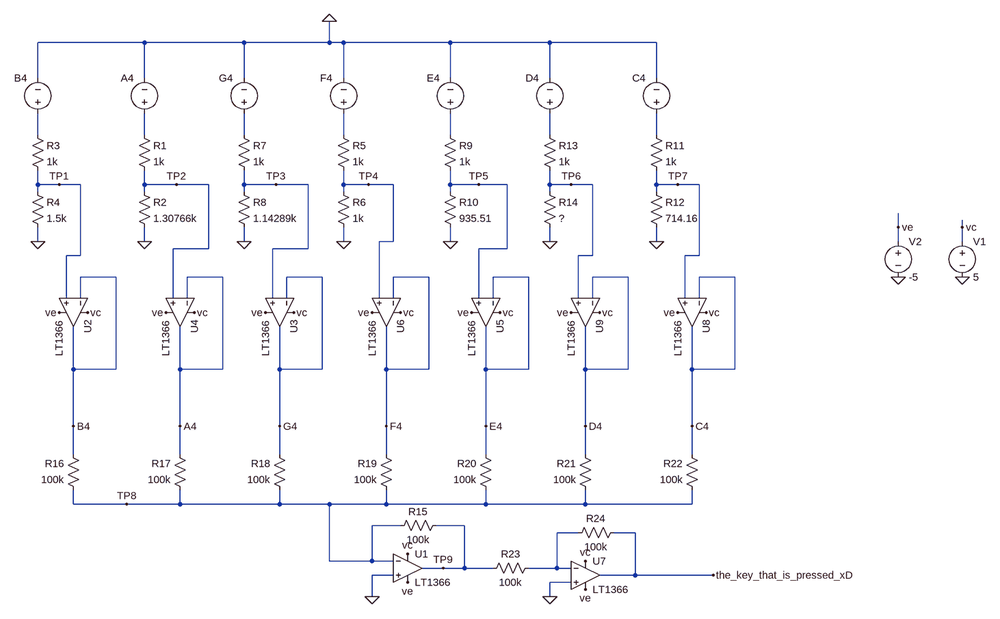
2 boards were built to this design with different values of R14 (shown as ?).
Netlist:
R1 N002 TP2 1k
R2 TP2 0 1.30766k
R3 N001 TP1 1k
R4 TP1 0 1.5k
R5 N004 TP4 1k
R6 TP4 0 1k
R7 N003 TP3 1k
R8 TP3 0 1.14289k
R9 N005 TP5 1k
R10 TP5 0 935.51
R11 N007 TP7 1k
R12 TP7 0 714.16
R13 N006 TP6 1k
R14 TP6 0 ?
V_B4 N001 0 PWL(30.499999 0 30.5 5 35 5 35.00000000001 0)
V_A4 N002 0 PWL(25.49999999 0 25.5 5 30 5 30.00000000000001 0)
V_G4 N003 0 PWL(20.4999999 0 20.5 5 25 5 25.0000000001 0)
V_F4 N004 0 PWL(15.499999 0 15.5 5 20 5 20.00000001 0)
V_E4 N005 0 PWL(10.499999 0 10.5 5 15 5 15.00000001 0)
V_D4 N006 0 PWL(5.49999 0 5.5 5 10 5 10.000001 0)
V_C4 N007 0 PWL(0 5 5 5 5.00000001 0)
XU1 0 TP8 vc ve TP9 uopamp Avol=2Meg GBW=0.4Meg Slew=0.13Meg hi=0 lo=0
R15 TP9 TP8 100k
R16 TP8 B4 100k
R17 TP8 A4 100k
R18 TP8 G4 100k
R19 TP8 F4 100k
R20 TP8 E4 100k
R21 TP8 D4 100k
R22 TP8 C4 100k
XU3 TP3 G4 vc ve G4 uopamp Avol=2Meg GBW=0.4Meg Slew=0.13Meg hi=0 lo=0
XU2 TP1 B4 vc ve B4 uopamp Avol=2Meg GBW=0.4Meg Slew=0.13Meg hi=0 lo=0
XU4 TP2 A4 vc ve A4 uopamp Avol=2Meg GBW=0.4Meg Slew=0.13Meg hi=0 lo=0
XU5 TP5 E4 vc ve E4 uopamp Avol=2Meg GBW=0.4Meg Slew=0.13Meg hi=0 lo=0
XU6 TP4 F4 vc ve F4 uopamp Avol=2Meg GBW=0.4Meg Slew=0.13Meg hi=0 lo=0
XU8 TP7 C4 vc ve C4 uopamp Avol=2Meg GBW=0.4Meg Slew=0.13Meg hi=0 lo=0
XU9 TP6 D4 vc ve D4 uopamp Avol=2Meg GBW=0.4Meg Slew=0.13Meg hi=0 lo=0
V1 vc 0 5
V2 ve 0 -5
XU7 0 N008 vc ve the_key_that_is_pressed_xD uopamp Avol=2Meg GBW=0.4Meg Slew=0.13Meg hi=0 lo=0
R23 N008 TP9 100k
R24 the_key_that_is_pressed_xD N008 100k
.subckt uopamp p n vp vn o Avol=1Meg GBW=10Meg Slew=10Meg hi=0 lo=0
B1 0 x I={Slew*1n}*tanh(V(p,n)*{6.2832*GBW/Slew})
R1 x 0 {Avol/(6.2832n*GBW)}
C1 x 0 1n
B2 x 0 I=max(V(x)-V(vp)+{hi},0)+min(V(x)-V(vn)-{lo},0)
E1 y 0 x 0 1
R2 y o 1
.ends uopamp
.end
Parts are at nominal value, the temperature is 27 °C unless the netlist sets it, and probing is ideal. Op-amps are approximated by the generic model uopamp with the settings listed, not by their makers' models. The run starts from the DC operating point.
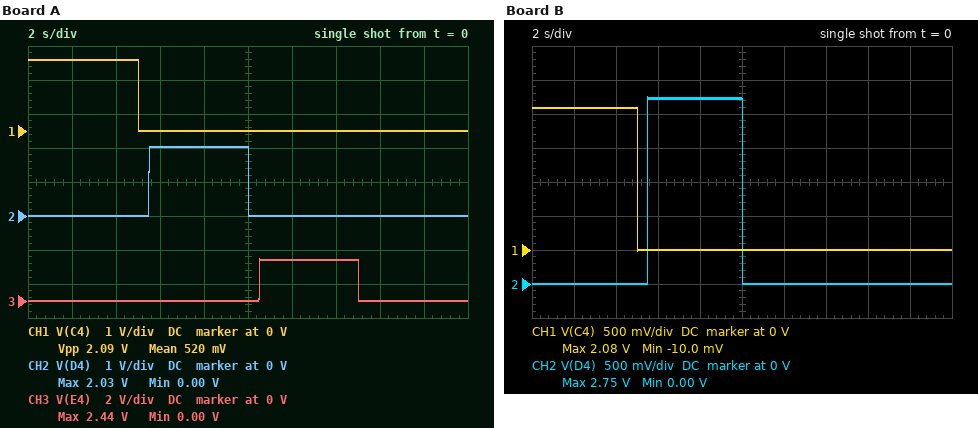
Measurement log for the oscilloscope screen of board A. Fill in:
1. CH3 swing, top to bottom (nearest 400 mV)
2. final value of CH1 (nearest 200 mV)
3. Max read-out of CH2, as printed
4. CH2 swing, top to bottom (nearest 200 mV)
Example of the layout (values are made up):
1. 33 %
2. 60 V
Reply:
1. 2.4 V
2. 0 V
3. 2.03 V
4. 2.0 V
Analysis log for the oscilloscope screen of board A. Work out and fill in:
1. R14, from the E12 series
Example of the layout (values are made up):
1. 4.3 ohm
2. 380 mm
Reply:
1. 680 Ω
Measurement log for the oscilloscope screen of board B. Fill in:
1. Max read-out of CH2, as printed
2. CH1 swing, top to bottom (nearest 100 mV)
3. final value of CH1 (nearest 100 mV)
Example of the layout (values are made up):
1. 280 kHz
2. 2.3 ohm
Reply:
1. 2.75 V
2. 2.1 V
3. 0 V
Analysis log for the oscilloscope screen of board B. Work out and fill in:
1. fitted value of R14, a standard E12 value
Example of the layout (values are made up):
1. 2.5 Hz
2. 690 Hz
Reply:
1. 1.2 kΩ
